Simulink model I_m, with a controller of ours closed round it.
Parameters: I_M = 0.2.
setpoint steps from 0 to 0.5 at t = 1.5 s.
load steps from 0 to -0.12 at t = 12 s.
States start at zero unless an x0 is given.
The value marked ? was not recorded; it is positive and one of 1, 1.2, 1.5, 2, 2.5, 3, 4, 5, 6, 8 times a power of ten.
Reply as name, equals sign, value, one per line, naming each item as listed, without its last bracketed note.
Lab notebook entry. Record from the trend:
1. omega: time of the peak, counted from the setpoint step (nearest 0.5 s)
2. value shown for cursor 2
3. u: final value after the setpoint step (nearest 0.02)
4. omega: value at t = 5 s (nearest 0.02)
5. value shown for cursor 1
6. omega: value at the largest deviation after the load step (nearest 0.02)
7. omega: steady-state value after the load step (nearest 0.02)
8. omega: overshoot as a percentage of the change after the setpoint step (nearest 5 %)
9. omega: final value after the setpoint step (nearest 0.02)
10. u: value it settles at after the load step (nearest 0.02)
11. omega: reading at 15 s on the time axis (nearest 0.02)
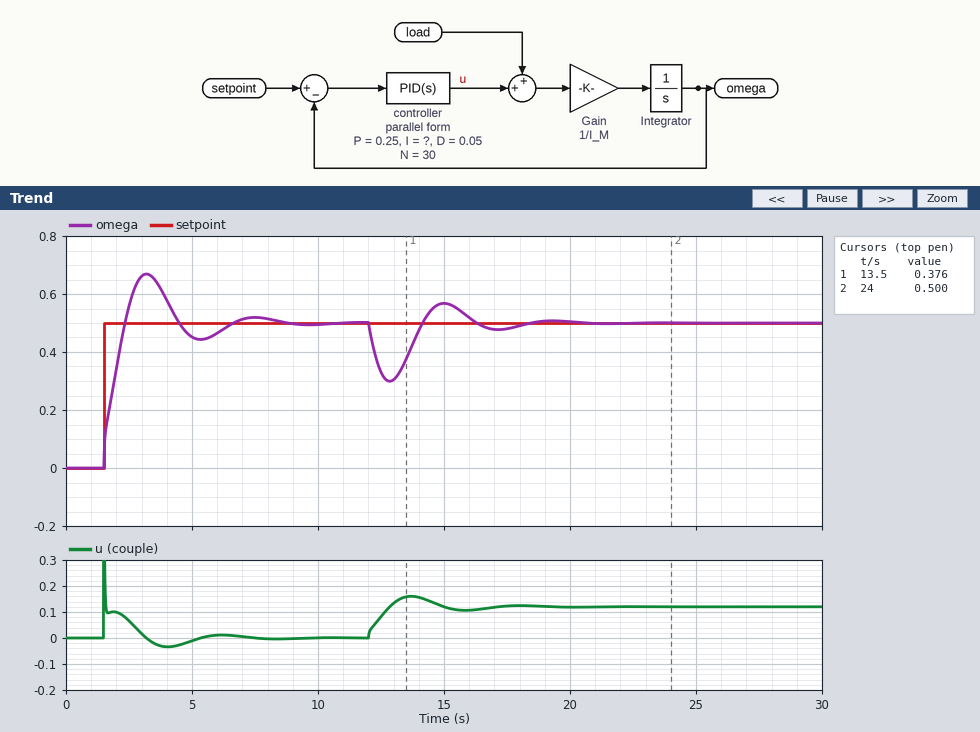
omega: time of the peak, counted from the setpoint step = 1.5 s
value shown for cursor 2 = 0.500
u: final value after the setpoint step = 0.00
omega: value at t = 5 s = 0.46
value shown for cursor 1 = 0.376
omega: value at the largest deviation after the load step = 0.30
omega: steady-state value after the load step = 0.50
omega: overshoot as a percentage of the change after the setpoint step = 35 %
omega: final value after the setpoint step = 0.50
u: value it settles at after the load step = 0.12
omega: reading at 15 s on the time axis = 0.56
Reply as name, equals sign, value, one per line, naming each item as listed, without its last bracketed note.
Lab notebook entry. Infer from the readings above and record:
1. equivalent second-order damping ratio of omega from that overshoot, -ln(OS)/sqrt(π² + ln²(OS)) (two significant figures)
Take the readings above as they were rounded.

equivalent second-order damping ratio of omega from that overshoot, -ln(OS)/sqrt(π² + ln²(OS)) = 0.32
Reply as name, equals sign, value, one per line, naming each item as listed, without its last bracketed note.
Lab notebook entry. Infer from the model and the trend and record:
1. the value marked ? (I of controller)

the value marked ? = 0.6
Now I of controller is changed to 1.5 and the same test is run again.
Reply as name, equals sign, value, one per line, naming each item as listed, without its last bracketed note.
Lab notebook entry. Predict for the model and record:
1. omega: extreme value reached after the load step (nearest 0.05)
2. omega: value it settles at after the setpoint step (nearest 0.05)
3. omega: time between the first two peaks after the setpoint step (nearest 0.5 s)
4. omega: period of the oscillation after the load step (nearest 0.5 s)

omega: extreme value reached after the load step = 0.35
omega: value it settles at after the setpoint step = 0.50
omega: time between the first two peaks after the setpoint step = 2.5 s
omega: period of the oscillation after the load step = 2.5 s
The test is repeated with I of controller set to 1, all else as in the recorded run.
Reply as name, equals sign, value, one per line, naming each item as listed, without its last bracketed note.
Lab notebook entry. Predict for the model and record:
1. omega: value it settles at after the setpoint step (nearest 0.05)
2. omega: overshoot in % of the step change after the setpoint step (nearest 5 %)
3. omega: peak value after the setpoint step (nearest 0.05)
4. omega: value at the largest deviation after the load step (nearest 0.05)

omega: value it settles at after the setpoint step = 0.50
omega: overshoot in % of the step change after the setpoint step = 40 %
omega: peak value after the setpoint step = 0.70
omega: value at the largest deviation after the load step = 0.35
